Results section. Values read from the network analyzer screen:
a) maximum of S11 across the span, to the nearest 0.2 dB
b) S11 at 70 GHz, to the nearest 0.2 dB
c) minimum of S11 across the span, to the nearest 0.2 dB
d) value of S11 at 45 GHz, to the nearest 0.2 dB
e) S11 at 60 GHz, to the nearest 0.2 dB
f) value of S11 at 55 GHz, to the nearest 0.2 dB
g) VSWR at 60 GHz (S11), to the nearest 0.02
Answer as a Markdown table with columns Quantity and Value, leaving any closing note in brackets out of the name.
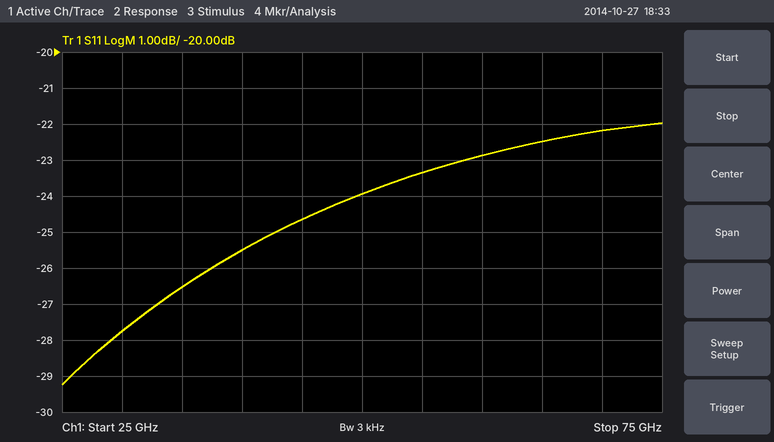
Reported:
| Quantity | Value |
|---|---|
| maximum of S11 across the span, to the nearest 0.2 dB | -22.0 dB |
| S11 at 70 GHz, to the nearest 0.2 dB | -22.2 dB |
| minimum of S11 across the span, to the nearest 0.2 dB | -29.2 dB |
| value of S11 at 45 GHz, to the nearest 0.2 dB | -24.6 dB |
| S11 at 60 GHz, to the nearest 0.2 dB | -22.8 dB |
| value of S11 at 55 GHz, to the nearest 0.2 dB | -23.4 dB |
| VSWR at 60 GHz (S11), to the nearest 0.02 | 1.16 |
